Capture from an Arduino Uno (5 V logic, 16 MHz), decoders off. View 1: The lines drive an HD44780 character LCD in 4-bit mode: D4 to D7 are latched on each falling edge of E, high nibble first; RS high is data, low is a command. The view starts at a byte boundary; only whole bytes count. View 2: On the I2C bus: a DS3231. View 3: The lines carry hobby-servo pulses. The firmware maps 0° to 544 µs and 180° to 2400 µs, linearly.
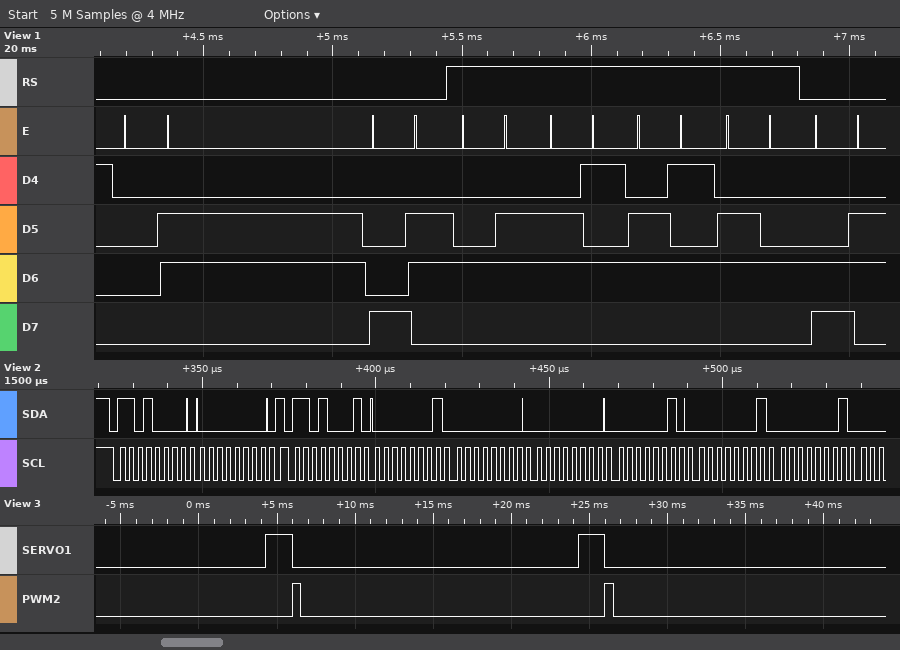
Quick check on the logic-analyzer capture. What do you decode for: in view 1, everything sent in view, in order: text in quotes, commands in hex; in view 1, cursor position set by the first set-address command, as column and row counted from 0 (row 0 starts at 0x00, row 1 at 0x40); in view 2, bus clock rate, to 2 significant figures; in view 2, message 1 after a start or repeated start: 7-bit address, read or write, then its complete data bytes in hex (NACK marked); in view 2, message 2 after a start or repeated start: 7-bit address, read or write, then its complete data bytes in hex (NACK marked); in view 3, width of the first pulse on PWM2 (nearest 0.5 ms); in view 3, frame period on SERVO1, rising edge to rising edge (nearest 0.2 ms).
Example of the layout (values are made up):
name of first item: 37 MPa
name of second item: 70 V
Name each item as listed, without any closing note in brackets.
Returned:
in view 1, everything sent in view, in order: text in quotes, commands in hex: 0x06 0x86 "Feed" 0xC6
in view 1, cursor position set by the first set-address command, as column and row counted from 0: column 6, row 0
in view 2, bus clock rate, to 2 significant figures: 400 kHz
in view 2, message 1 after a start or repeated start: 7-bit address, read or write, then its complete data bytes in hex: 0x68 write: 00
in view 2, message 2 after a start or repeated start: 7-bit address, read or write, then its complete data bytes in hex: 0x68 read: 01 00 00 02 01 01
in view 3, width of the first pulse on PWM2: 0.5 ms
in view 3, frame period on SERVO1, rising edge to rising edge: 20.0 ms
